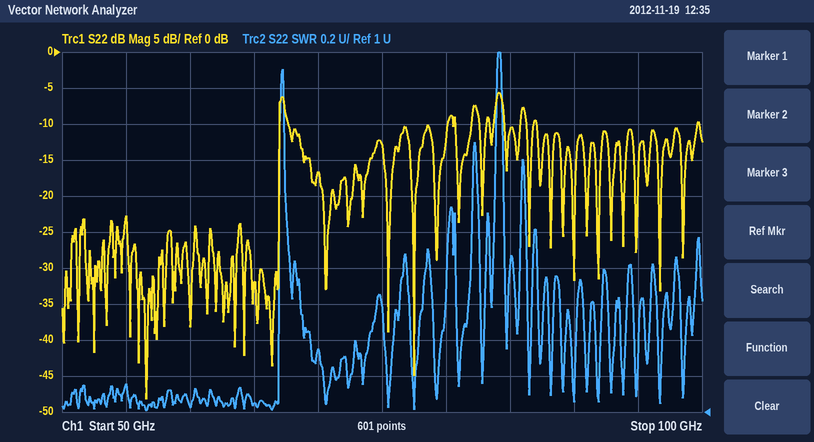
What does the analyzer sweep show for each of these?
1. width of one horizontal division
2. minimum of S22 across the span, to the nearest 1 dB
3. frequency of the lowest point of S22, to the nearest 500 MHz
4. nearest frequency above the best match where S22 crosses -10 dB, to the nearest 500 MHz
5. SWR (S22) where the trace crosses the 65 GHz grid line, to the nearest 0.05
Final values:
5 GHz
-48 dB
56.5 GHz
67.0 GHz
1.05
